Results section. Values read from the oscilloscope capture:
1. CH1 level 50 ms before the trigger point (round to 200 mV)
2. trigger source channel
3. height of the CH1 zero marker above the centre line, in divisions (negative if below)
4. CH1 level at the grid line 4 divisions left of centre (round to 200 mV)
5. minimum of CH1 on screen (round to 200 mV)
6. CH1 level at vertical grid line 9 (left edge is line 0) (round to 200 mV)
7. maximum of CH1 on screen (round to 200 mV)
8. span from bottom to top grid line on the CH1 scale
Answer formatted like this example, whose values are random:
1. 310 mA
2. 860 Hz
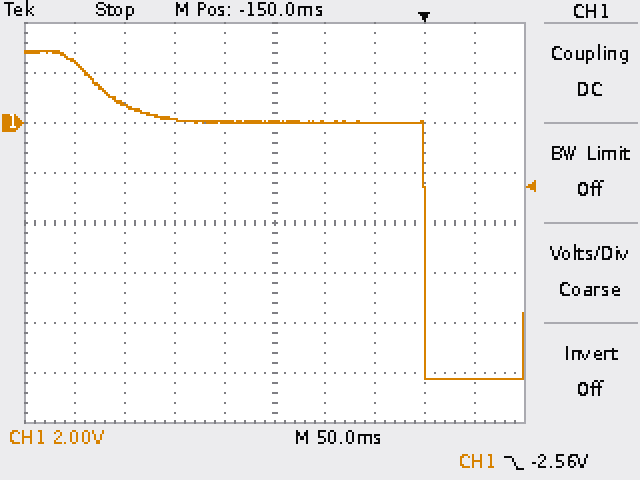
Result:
1. 0.0 V
2. CH1
3. +2.0 div
4. 2.4 V
5. -10.2 V
6. -10.2 V
7. 2.8 V
8. 16 V
